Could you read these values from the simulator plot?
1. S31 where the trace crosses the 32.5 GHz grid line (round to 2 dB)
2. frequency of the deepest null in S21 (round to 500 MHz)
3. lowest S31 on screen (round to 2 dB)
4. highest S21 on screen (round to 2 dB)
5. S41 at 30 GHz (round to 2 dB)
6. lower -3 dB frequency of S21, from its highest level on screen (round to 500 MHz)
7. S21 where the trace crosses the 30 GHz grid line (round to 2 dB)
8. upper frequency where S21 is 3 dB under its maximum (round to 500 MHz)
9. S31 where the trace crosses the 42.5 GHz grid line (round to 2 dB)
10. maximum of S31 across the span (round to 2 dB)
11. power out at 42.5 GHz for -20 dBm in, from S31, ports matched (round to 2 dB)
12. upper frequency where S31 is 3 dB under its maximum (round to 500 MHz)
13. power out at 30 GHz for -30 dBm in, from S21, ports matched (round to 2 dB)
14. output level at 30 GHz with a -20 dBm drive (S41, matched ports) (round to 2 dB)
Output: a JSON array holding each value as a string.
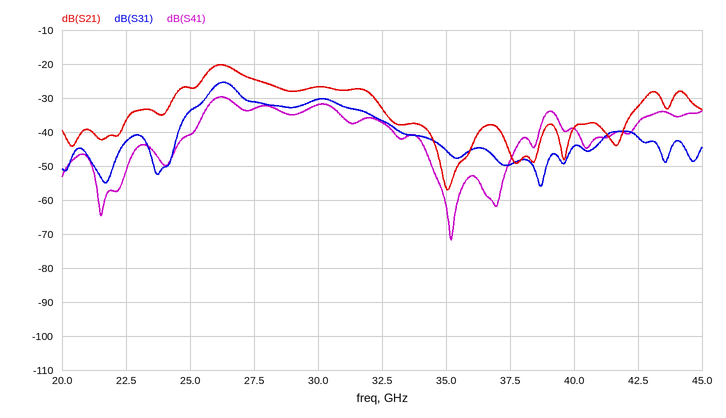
["-36 dB", "35.0 GHz", "-56 dB", "-20 dB", "-32 dB", "25.5 GHz", "-26 dB", "27.0 GHz", "-42 dB", "-26 dB", "-62 dBm", "27.0 GHz", "-56 dBm", "-52 dBm"]
